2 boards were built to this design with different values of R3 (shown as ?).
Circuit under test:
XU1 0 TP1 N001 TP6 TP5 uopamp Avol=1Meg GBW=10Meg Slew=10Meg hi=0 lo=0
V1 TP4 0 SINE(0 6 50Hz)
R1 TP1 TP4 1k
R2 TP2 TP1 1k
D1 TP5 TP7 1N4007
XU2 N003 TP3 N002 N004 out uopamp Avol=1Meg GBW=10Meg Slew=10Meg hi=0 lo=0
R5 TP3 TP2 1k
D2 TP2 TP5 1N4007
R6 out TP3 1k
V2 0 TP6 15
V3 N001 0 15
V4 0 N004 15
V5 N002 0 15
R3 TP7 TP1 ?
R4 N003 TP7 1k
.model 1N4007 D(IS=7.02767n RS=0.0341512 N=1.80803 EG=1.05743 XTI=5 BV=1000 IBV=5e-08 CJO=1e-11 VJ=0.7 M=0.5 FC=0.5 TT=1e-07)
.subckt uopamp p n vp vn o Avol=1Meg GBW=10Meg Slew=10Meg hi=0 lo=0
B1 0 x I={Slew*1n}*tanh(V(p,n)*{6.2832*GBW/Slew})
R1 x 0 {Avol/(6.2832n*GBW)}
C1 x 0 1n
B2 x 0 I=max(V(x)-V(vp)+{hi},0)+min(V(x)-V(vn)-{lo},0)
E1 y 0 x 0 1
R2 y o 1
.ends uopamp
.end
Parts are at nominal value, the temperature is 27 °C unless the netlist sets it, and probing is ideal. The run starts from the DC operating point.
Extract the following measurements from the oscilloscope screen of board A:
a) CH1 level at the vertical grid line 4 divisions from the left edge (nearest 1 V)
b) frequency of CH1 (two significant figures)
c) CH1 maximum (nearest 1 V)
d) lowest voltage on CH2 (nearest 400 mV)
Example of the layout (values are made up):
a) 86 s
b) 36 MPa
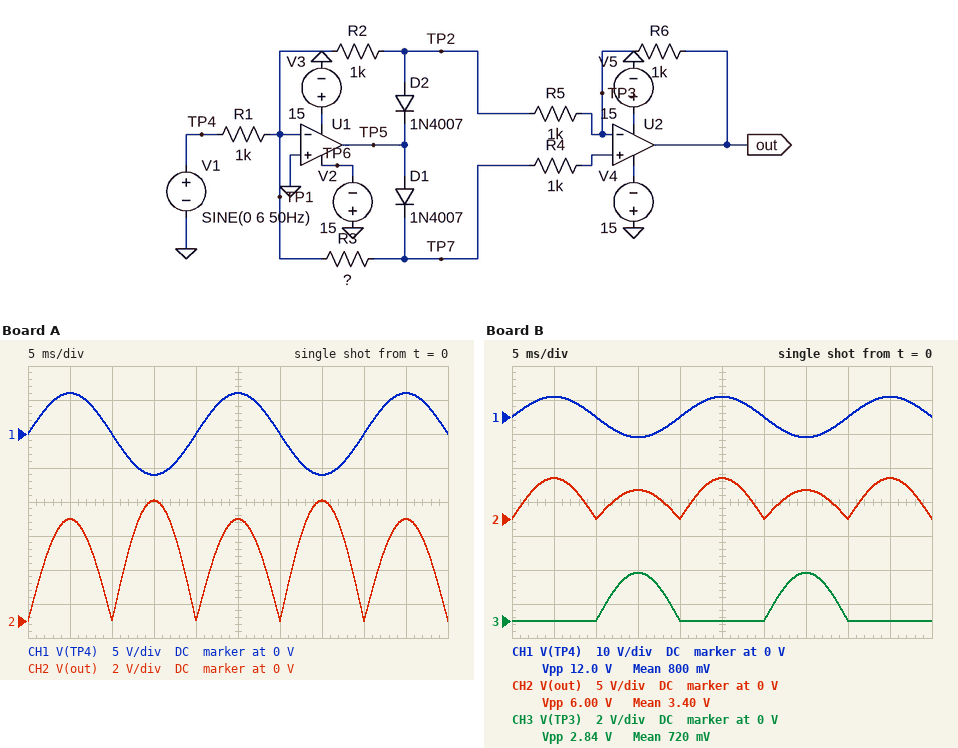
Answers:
a) 0 V
b) 50 Hz
c) 6 V
d) 0 V
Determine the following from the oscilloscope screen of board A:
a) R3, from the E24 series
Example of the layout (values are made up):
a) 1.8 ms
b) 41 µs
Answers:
a) 1.3 kΩ
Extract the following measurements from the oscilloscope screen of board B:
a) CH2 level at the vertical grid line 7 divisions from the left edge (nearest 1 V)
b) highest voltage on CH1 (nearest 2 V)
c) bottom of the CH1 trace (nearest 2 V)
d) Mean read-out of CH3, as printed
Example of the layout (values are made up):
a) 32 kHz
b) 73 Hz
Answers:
a) 4 V
b) 6 V
c) -6 V
d) 720 mV
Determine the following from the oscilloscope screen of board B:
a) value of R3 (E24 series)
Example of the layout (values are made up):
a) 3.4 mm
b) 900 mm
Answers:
a) 620 Ω
